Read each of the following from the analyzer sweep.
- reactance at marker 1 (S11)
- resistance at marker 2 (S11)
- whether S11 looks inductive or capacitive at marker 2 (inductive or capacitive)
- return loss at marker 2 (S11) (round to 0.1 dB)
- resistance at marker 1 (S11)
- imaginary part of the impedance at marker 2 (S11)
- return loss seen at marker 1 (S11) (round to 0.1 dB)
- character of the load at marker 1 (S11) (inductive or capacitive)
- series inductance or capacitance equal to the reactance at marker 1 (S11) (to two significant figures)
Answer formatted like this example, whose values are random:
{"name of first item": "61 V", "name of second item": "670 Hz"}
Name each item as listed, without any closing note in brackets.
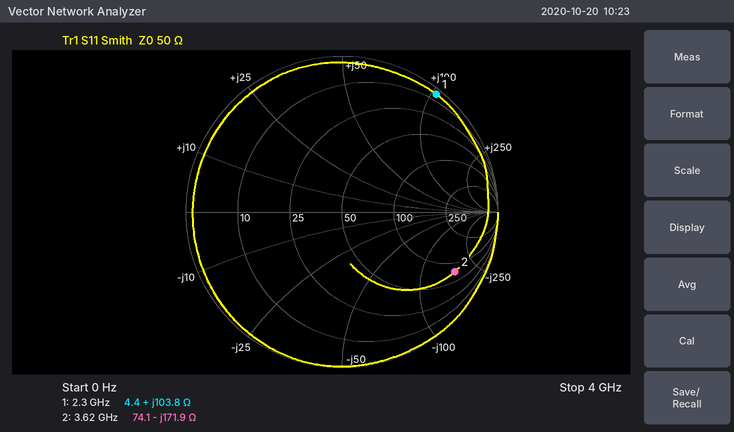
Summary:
{"reactance at marker 1": "+103.8 Ω", "resistance at marker 2": "74.1 Ω", "whether S11 looks inductive or capacitive at marker 2": "capacitive", "return loss at marker 2 (S11)": "1.7 dB", "resistance at marker 1": "4.4 Ω", "imaginary part of the impedance at marker 2": "-171.9 Ω", "return loss seen at marker 1 (S11)": "0.3 dB", "character of the load at marker 1 (S11)": "inductive", "series inductance or capacitance equal to the reactance at marker 1 (S11)": "7.2 nH"}
